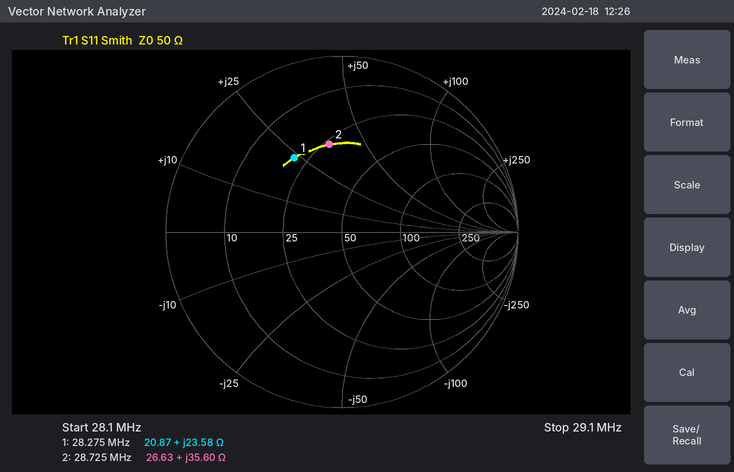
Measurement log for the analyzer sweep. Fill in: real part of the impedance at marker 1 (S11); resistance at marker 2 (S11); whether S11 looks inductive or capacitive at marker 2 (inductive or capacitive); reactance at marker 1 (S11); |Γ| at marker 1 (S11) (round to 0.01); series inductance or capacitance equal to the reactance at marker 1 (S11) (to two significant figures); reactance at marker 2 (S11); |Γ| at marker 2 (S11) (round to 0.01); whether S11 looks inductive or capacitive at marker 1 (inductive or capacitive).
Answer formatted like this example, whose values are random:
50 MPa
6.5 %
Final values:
20.87 Ω
26.63 Ω
inductive
+23.58 Ω
0.50
130 nH
+35.60 Ω
0.50
inductive
